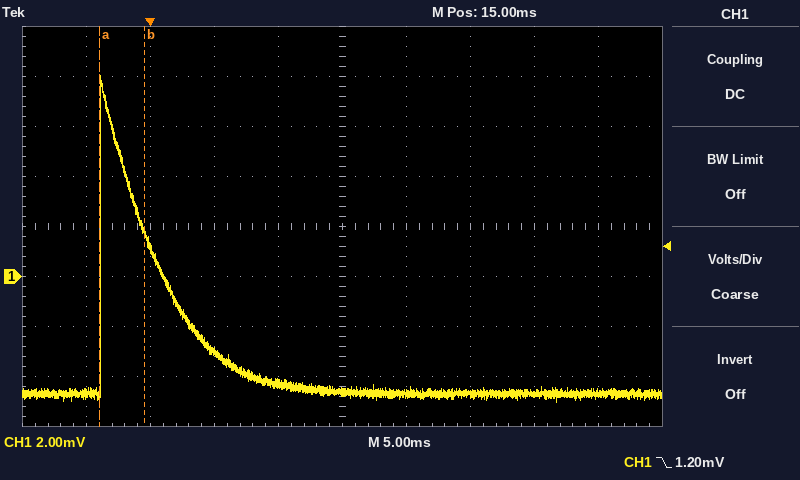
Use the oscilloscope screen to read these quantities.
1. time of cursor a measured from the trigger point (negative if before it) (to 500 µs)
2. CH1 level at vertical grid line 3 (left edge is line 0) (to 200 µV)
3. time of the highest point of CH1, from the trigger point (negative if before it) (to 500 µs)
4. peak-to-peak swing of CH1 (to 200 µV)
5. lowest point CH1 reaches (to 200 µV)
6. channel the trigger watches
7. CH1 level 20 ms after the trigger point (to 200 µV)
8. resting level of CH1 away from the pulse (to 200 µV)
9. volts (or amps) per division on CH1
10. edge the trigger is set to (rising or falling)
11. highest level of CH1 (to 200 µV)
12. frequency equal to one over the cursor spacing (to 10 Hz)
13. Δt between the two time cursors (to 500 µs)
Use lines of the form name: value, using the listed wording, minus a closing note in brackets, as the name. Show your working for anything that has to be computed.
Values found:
time of cursor a measured from the trigger point (negative if before it): -4.0 ms
CH1 level at vertical grid line 3 (left edge is line 0): -3.0 mV
time of the highest point of CH1, from the trigger point (negative if before it): -4.0 ms
peak-to-peak swing of CH1: 8.0 mV − (-5.0 mV) = 13.0 mV
lowest point CH1 reaches: -5.0 mV
channel the trigger watches: CH1
CH1 level 20 ms after the trigger point: -4.6 mV
resting level of CH1 away from the pulse: -4.6 mV
volts (or amps) per division on CH1: 2 mV
edge the trigger is set to: falling
highest level of CH1: 8.0 mV
frequency equal to one over the cursor spacing: 1 / 3.5 ms ≈ 290 Hz
Δt between the two time cursors: 3.5 ms
